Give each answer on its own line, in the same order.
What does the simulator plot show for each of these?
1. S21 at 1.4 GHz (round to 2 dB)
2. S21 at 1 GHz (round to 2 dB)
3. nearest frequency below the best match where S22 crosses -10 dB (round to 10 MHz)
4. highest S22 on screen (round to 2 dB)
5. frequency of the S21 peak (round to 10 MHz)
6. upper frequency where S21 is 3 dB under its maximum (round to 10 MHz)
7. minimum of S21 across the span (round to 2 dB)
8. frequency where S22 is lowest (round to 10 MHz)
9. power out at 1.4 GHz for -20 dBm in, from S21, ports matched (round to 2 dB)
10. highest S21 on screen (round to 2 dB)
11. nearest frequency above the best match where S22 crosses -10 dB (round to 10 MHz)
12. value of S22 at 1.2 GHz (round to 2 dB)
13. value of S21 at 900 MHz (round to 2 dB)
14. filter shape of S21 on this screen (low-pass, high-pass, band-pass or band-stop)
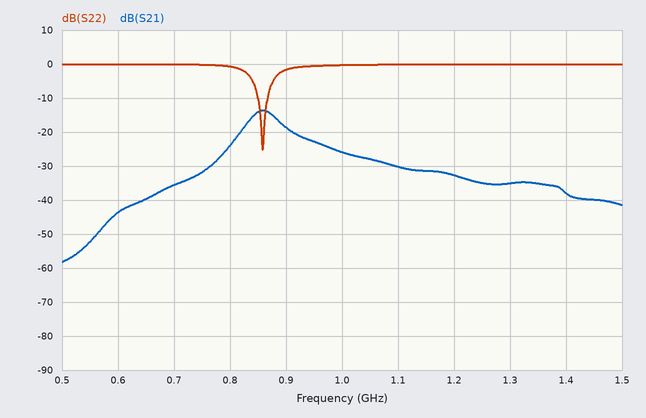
-38 dB
-26 dB
850 MHz
0 dB
860 MHz
890 MHz
-58 dB
860 MHz
-58 dBm
-14 dB
870 MHz
0 dB
-18 dB
band-pass
